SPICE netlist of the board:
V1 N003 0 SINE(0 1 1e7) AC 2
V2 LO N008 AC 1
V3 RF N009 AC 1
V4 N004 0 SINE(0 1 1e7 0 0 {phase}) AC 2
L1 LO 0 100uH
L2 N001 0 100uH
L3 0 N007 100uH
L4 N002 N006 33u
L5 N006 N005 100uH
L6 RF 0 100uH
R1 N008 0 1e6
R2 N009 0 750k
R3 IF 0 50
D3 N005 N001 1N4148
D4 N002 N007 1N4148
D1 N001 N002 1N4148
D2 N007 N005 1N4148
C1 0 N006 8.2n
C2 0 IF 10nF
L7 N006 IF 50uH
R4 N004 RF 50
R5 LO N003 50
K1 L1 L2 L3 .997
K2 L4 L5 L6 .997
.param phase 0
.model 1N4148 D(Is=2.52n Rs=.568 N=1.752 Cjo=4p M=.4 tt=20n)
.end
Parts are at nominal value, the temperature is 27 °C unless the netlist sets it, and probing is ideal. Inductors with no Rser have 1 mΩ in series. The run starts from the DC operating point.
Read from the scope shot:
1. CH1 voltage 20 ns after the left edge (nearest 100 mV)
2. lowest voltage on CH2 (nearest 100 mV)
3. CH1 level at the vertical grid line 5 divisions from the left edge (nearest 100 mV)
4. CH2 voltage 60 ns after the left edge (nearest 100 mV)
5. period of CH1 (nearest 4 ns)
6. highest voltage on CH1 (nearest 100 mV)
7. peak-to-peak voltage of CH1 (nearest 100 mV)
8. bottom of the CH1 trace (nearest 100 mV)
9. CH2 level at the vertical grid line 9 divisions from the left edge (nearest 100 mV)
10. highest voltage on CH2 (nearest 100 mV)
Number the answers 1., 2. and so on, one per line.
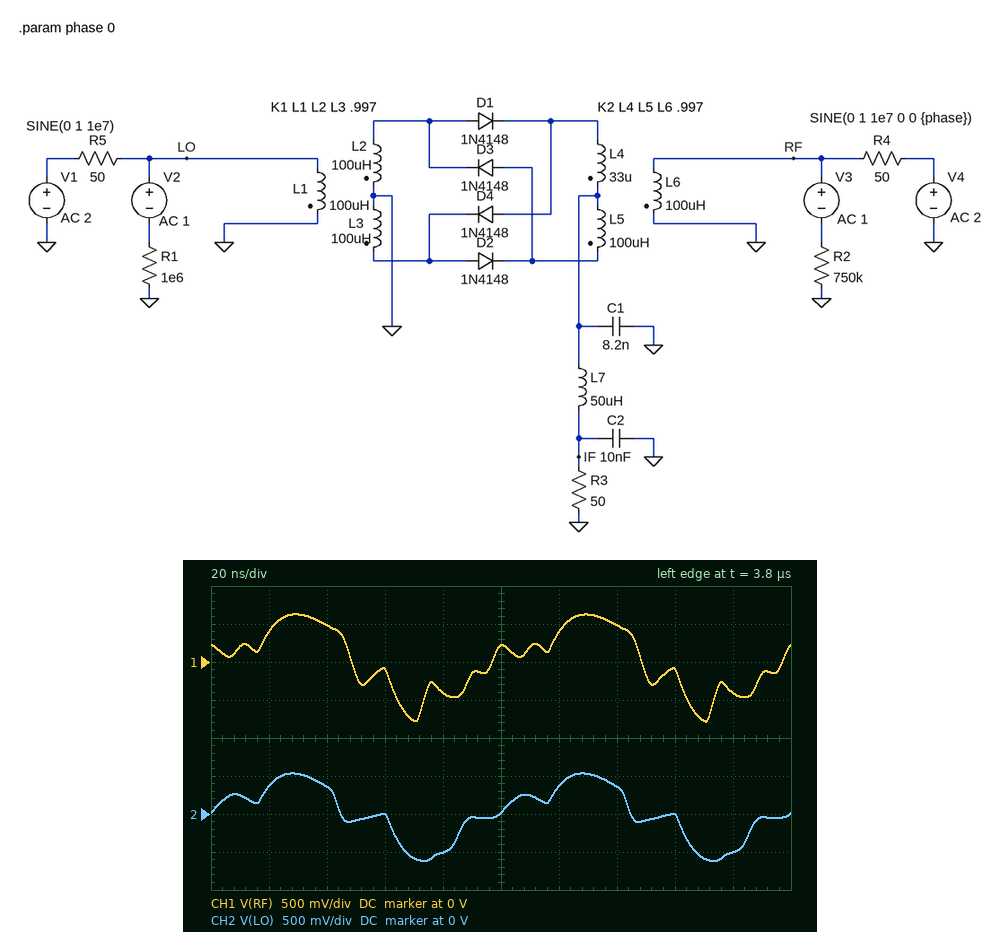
1. 400 mV
2. -600 mV
3. 200 mV
4. 0 V
5. 100 ns
6. 600 mV
7. 1.4 V
8. -800 mV
9. -500 mV
10. 500 mV
